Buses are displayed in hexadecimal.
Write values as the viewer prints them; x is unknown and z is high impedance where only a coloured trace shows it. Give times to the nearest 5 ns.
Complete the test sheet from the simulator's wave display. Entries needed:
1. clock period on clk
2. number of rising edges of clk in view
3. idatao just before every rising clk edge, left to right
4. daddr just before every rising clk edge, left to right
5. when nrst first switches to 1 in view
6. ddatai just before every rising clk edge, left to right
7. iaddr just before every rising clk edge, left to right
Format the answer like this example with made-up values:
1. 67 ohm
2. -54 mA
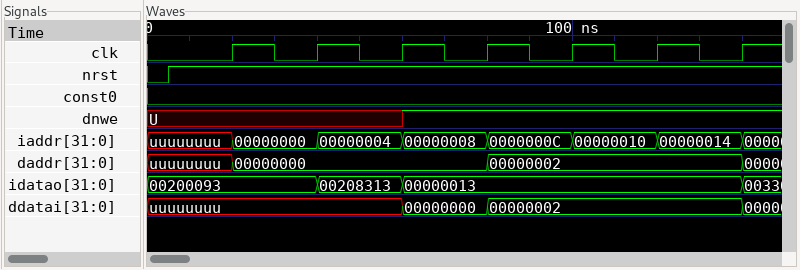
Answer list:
1. 20 ns
2. 7
3. 00200093, 00200093, 00208313, 00000013, 00000013, 00000013, 00000013
4. uuuuuuuu, 00000000, 00000000, 00000000, 00000002, 00000002, 00000002
5. 5 ns
6. uuuuuuuu, uuuuuuuu, uuuuuuuu, 00000000, 00000002, 00000002, 00000002
7. uuuuuuuu, 00000000, 00000004, 00000008, 0000000C, 00000010, 00000014
